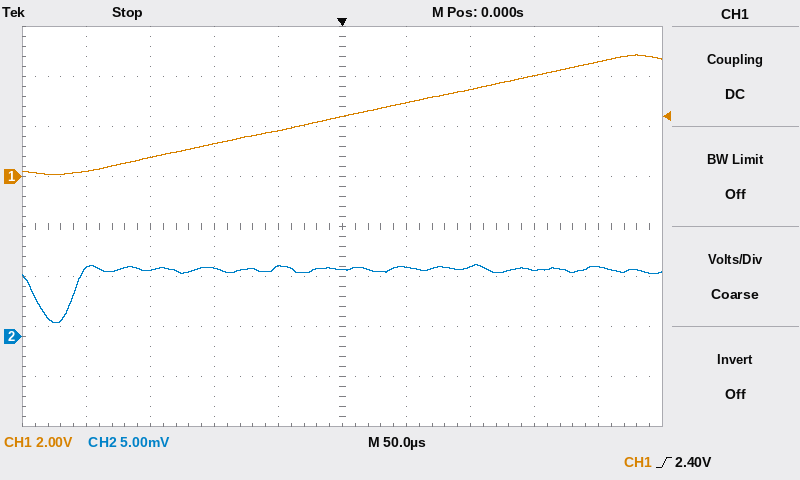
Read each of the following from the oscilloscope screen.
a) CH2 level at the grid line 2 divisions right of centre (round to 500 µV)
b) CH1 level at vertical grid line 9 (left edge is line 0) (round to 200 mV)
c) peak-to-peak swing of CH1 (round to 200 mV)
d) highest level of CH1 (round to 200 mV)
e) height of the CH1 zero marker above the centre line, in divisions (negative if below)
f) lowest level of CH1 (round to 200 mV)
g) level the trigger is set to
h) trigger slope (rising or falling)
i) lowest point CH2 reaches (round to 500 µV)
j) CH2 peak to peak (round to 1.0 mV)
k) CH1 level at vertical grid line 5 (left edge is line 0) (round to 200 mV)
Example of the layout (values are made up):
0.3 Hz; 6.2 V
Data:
7.0 mV; 4.6 V; 4.8 V; 4.8 V; +1.0 div; 0.0 V; 2.40 V; rising; 1.5 mV; 6.0 mV; 2.4 V
